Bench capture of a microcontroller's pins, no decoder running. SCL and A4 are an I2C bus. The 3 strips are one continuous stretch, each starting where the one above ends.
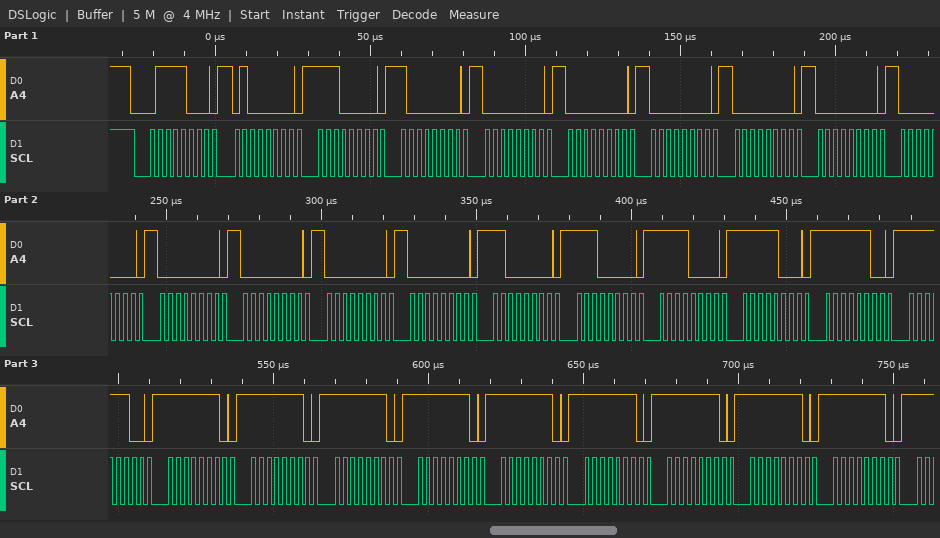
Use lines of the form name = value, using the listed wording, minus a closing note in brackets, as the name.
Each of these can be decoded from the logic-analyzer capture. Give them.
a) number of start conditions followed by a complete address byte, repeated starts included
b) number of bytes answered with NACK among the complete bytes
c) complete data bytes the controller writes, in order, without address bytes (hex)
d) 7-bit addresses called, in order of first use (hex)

number of start conditions followed by a complete address byte, repeated starts included = 1
number of bytes answered with NACK among the complete bytes = 0
complete data bytes the controller writes, in order, without address bytes = 40 E0 80 00 00 00 00 00 00 00 00 00 00 C0 E0 F0 F8 FC FC FE FE FE FE FE FE FE FE FE
7-bit addresses called, in order of first use = 0x3C
